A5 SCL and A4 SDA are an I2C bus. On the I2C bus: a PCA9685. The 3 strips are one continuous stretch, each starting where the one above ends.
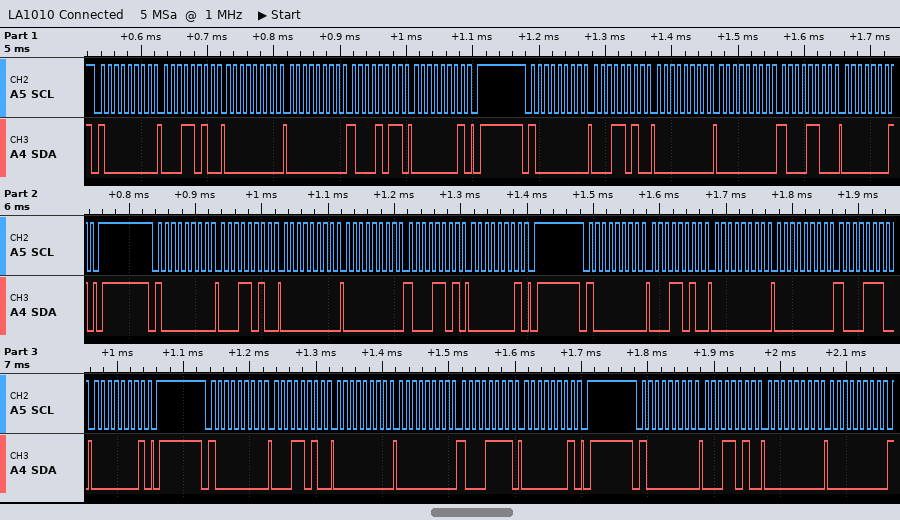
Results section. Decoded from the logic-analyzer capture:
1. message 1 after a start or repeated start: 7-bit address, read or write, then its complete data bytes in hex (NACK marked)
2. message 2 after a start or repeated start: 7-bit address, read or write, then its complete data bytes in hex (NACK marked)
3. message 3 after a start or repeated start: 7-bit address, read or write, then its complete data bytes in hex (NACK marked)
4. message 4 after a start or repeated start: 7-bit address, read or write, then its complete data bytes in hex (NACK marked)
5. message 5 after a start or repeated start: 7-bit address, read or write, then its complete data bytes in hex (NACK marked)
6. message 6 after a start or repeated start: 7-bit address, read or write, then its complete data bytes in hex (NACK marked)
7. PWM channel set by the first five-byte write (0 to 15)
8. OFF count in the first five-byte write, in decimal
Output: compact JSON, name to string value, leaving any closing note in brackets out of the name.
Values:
{"message 1 after a start or repeated start: 7-bit address, read or write, then its complete data bytes in hex": "0x40 write: 1A 00 00 8B 01", "message 2 after a start or repeated start: 7-bit address, read or write, then its complete data bytes in hex": "0x40 write: 1A 00 00 8C 01", "message 3 after a start or repeated start: 7-bit address, read or write, then its complete data bytes in hex": "0x40 write: 1A 00 00 8D 01", "message 4 after a start or repeated start: 7-bit address, read or write, then its complete data bytes in hex": "0x40 write: 1A 00 00 8E 01", "message 5 after a start or repeated start: 7-bit address, read or write, then its complete data bytes in hex": "0x40 write: 1A 00 00 8F 01", "message 6 after a start or repeated start: 7-bit address, read or write, then its complete data bytes in hex": "0x40 write: 1A 00 00", "PWM channel set by the first five-byte write": "5", "OFF count in the first five-byte write, in decimal": "395"}
